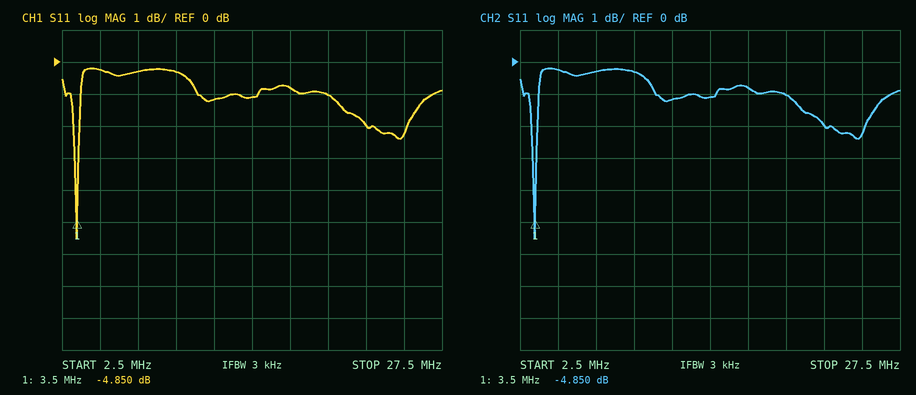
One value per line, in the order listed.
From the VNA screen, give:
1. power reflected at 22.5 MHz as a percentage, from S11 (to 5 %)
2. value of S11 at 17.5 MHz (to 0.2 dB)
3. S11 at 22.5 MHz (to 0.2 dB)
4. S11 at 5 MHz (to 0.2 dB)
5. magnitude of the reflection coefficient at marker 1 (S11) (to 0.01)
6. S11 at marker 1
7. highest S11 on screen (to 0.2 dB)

65 %
-0.8 dB
-2.0 dB
-0.2 dB
0.57
-4.850 dB
-0.2 dB
